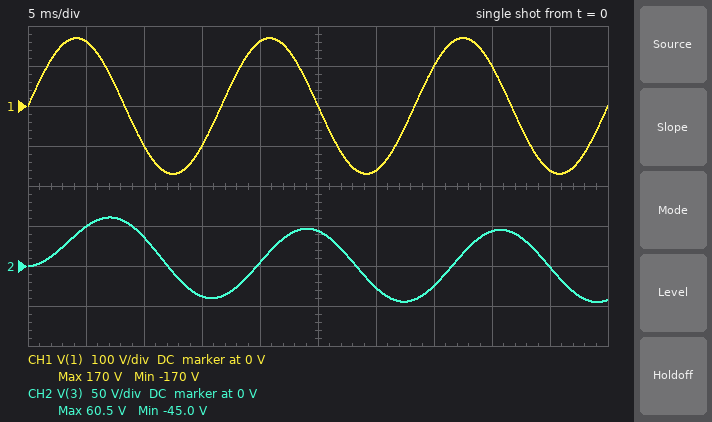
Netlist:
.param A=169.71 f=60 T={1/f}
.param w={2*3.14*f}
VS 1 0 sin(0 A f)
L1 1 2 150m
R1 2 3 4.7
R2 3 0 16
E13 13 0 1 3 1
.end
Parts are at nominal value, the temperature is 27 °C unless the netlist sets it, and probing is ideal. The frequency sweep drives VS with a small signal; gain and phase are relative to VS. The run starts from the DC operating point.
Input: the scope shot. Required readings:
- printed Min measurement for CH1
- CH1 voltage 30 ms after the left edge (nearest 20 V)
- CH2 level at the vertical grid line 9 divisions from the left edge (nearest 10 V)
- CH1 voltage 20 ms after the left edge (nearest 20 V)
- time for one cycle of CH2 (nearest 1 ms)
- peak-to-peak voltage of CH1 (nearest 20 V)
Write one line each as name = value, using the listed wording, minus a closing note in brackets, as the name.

printed Min measurement for CH1 = -170 V
CH1 voltage 30 ms after the left edge = -160 V
CH2 level at the vertical grid line 9 divisions from the left edge = 0 V
CH1 voltage 20 ms after the left edge = 160 V
time for one cycle of CH2 = 17 ms
peak-to-peak voltage of CH1 = 340 V
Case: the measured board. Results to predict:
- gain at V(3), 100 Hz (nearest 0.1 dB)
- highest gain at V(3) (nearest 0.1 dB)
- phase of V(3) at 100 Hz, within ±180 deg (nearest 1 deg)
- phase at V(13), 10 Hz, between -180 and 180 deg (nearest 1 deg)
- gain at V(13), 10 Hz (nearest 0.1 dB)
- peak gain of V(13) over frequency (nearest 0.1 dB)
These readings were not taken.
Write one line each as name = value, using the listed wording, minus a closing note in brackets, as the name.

gain at V(3), 100 Hz = -15.6 dB
highest gain at V(3) = -2.2 dB
phase of V(3) at 100 Hz, within ±180 deg = -78 deg
phase at V(13), 10 Hz, between -180 and 180 deg = 39 deg
gain at V(13), 10 Hz = -6.7 dB
peak gain of V(13) over frequency = 0 dB
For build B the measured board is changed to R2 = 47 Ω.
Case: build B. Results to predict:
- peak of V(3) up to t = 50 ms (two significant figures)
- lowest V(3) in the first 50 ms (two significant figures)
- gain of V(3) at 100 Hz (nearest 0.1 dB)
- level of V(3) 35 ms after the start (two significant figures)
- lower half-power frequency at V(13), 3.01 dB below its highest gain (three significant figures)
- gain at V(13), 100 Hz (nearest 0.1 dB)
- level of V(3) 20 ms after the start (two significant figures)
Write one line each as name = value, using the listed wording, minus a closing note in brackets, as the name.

peak of V(3) up to t = 50 ms = 110 V
lowest V(3) in the first 50 ms = -100 V
gain of V(3) at 100 Hz = -7.2 dB
level of V(3) 35 ms after the start = -21 V
lower half-power frequency at V(13), 3.01 dB below its highest gain = 54.4 Hz
gain at V(13), 100 Hz = -1.1 dB
level of V(3) 20 ms after the start = 43 V
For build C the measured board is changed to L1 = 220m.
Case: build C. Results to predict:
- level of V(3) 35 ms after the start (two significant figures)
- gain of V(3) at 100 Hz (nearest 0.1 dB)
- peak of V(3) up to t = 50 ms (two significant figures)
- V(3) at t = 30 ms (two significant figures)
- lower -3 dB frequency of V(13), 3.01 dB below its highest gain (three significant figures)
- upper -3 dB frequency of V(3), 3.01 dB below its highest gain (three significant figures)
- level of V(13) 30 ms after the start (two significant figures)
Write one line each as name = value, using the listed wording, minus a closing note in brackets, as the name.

level of V(3) 35 ms after the start = -19 V
gain of V(3) at 100 Hz = -18.8 dB
peak of V(3) up to t = 50 ms = 47 V
V(3) at t = 30 ms = -15 V
lower -3 dB frequency of V(13), 3.01 dB below its highest gain = 14.2 Hz
upper -3 dB frequency of V(3), 3.01 dB below its highest gain = 15.0 Hz
level of V(13) 30 ms after the start = -150 V
